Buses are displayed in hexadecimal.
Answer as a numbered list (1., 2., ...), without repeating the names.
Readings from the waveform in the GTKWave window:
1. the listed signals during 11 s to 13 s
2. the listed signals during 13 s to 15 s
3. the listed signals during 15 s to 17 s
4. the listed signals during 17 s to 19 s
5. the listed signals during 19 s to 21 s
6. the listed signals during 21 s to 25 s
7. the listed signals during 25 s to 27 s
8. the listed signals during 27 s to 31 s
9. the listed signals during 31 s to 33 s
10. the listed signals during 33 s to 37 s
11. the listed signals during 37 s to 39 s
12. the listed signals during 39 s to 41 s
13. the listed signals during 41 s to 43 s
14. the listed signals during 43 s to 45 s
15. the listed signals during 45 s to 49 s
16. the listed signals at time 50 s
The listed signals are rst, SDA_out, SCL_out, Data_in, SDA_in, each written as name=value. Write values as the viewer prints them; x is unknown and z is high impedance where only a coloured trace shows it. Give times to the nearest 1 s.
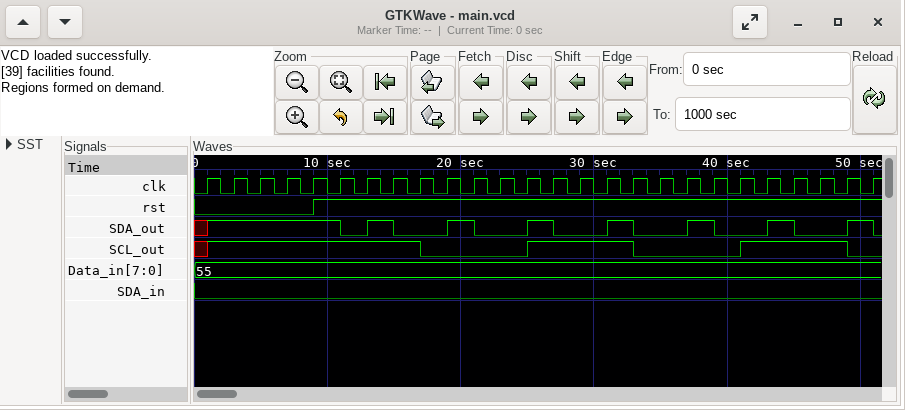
1. rst=1, SDA_out=0, SCL_out=1, Data_in=55, SDA_in=0
2. rst=1, SDA_out=1, SCL_out=1, Data_in=55, SDA_in=0
3. rst=1, SDA_out=0, SCL_out=1, Data_in=55, SDA_in=0
4. rst=1, SDA_out=0, SCL_out=0, Data_in=55, SDA_in=0
5. rst=1, SDA_out=1, SCL_out=0, Data_in=55, SDA_in=0
6. rst=1, SDA_out=0, SCL_out=0, Data_in=55, SDA_in=0
7. rst=1, SDA_out=1, SCL_out=1, Data_in=55, SDA_in=0
8. rst=1, SDA_out=0, SCL_out=1, Data_in=55, SDA_in=0
9. rst=1, SDA_out=1, SCL_out=1, Data_in=55, SDA_in=0
10. rst=1, SDA_out=0, SCL_out=0, Data_in=55, SDA_in=0
11. rst=1, SDA_out=1, SCL_out=0, Data_in=55, SDA_in=0
12. rst=1, SDA_out=0, SCL_out=0, Data_in=55, SDA_in=0
13. rst=1, SDA_out=0, SCL_out=1, Data_in=55, SDA_in=0
14. rst=1, SDA_out=1, SCL_out=1, Data_in=55, SDA_in=0
15. rst=1, SDA_out=0, SCL_out=1, Data_in=55, SDA_in=0
16. rst=1, SDA_out=1, SCL_out=0, Data_in=55, SDA_in=0
